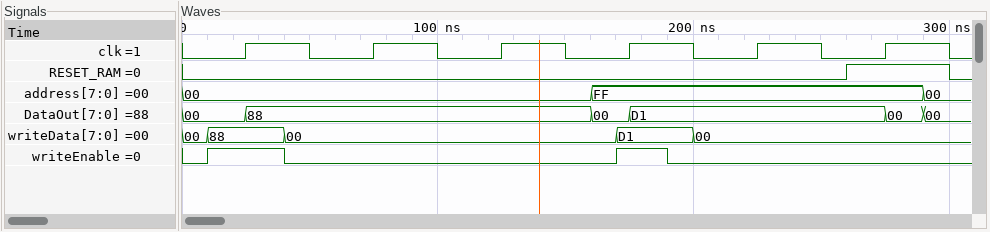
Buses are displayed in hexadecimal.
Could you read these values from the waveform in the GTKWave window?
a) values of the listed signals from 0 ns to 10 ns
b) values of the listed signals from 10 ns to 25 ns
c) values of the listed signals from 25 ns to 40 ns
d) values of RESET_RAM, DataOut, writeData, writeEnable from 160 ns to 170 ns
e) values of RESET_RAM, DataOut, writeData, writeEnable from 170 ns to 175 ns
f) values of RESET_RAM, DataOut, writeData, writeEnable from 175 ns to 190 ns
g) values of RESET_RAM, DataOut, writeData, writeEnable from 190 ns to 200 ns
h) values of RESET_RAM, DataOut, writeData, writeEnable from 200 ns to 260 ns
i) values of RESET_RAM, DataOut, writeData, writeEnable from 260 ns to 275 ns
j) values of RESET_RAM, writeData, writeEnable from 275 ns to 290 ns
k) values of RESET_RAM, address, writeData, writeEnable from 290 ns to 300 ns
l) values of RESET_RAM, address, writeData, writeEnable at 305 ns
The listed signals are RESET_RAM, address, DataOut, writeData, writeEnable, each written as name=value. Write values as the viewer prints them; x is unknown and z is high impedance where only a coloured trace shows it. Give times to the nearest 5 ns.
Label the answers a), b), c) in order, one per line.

a) RESET_RAM=0, address=00, DataOut=00, writeData=00, writeEnable=0
b) RESET_RAM=0, address=00, DataOut=00, writeData=88, writeEnable=1
c) RESET_RAM=0, address=00, DataOut=88, writeData=88, writeEnable=1
d) RESET_RAM=0, DataOut=00, writeData=00, writeEnable=0
e) RESET_RAM=0, DataOut=00, writeData=D1, writeEnable=1
f) RESET_RAM=0, DataOut=D1, writeData=D1, writeEnable=1
g) RESET_RAM=0, DataOut=D1, writeData=D1, writeEnable=0
h) RESET_RAM=0, DataOut=D1, writeData=00, writeEnable=0
i) RESET_RAM=1, DataOut=D1, writeData=00, writeEnable=0
j) RESET_RAM=1, writeData=00, writeEnable=0
k) RESET_RAM=1, address=00, writeData=00, writeEnable=0
l) RESET_RAM=0, address=00, writeData=00, writeEnable=0
